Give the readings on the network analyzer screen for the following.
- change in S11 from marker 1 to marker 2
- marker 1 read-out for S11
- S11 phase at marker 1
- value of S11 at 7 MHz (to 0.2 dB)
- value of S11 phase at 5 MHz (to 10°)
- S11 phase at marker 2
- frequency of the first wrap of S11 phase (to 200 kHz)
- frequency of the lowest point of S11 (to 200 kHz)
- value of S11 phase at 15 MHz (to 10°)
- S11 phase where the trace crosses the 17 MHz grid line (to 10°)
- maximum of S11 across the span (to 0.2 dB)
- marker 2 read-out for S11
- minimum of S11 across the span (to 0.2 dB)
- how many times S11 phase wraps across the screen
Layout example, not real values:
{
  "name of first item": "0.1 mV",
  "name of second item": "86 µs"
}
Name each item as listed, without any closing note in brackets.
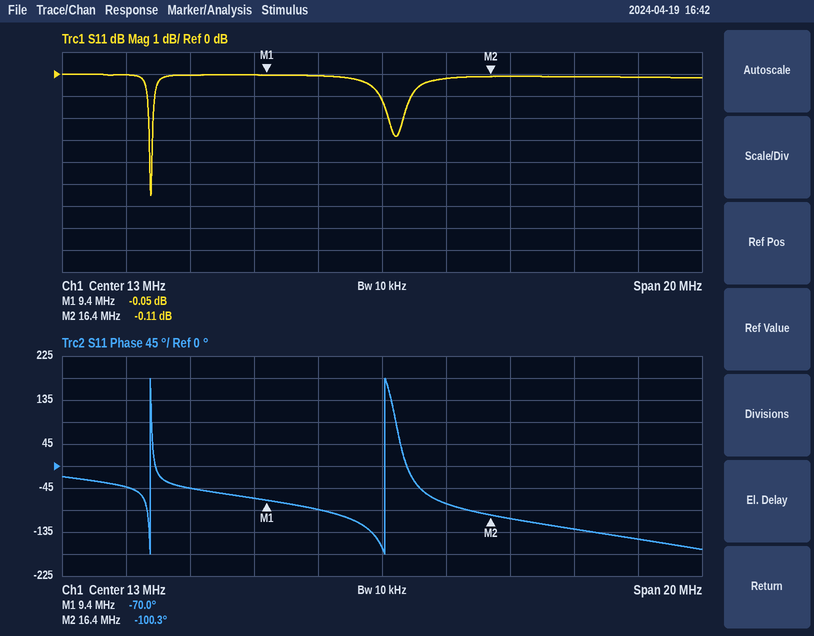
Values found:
{
  "change in S11 from marker 1 to marker 2": "-0.06 dB",
  "marker 1 read-out for S11": "-0.05 dB",
  "S11 phase at marker 1": "-70.0°",
  "value of S11 at 7 MHz": "0.0 dB",
  "value of S11 phase at 5 MHz": "-40°",
  "S11 phase at marker 2": "-100.3°",
  "frequency of the first wrap of S11 phase": "5.8 MHz",
  "frequency of the lowest point of S11": "5.8 MHz",
  "value of S11 phase at 15 MHz": "-80°",
  "S11 phase where the trace crosses the 17 MHz grid line": "-110°",
  "maximum of S11 across the span": "0.0 dB",
  "marker 2 read-out for S11": "-0.11 dB",
  "minimum of S11 across the span": "-5.6 dB",
  "how many times S11 phase wraps across the screen": "2"
}
